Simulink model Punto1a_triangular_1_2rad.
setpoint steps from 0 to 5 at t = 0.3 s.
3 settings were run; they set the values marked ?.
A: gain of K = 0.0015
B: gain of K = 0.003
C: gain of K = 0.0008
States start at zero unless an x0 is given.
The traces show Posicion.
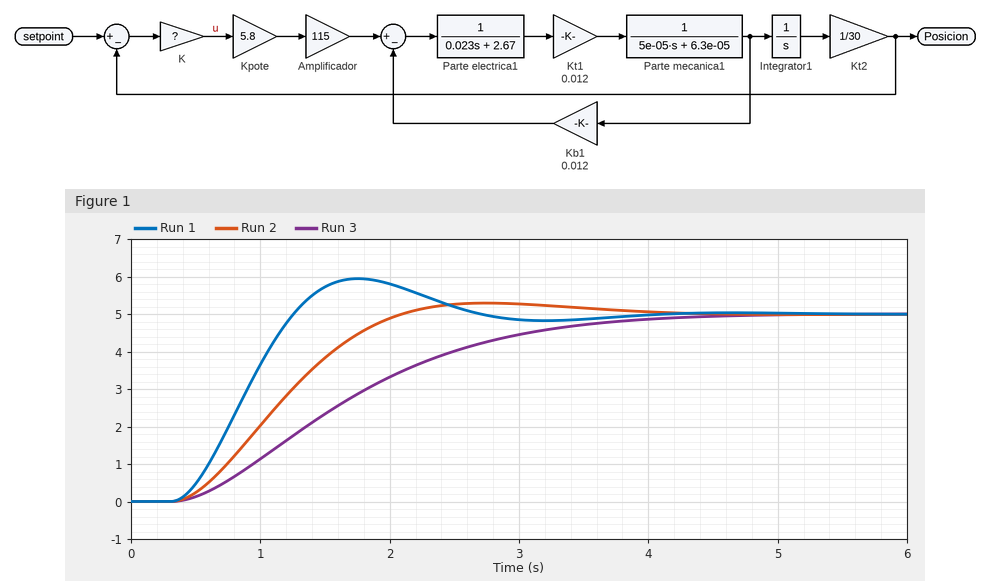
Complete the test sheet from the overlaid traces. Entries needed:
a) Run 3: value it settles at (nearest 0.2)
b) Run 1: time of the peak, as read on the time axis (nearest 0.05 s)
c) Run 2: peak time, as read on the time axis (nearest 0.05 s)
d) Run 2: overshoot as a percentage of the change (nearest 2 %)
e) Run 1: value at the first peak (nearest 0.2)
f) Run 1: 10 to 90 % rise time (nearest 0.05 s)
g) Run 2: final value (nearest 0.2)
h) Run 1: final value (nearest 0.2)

5.0
1.75 s
2.75 s
6 %
6.0
0.65 s
5.0
5.0
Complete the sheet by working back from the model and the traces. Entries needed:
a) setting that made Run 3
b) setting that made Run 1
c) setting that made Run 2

C
B
A
